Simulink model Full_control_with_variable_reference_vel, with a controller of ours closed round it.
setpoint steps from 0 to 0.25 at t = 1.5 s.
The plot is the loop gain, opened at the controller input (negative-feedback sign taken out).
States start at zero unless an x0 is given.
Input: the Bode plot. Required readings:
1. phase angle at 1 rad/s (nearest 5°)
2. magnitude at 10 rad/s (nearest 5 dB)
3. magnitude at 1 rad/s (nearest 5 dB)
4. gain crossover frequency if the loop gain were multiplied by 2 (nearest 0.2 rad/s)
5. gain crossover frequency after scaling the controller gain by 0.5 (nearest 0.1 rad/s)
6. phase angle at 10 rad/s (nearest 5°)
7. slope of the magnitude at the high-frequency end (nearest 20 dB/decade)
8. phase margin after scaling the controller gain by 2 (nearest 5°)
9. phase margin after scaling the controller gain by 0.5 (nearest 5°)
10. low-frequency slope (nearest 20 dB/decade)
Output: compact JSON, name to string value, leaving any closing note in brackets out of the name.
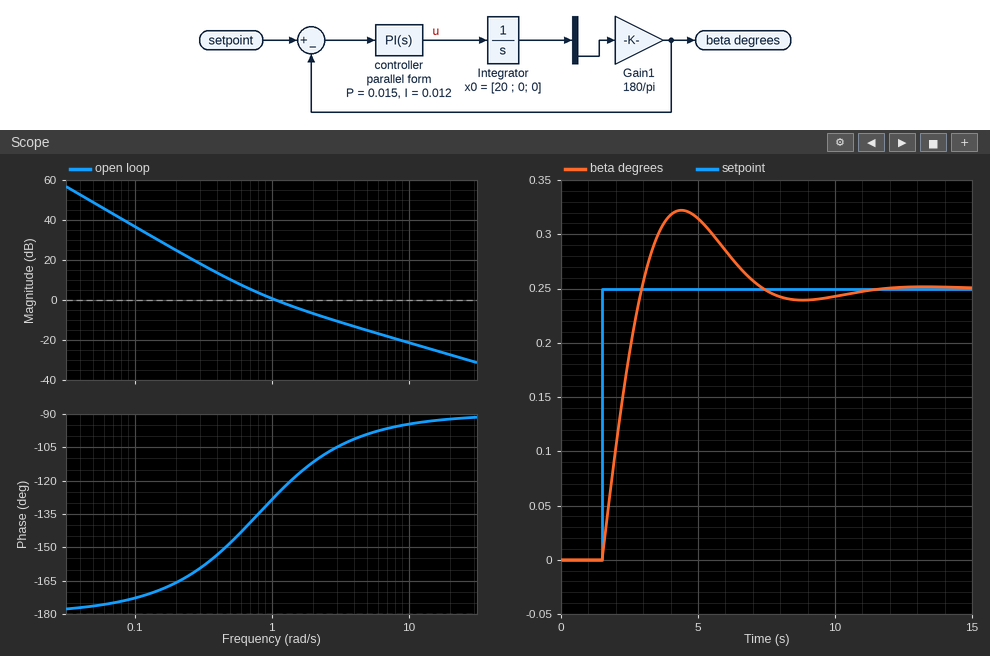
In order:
{"phase angle at 1 rad/s": "-130°", "magnitude at 10 rad/s": "-20 dB", "magnitude at 1 rad/s": "0 dB", "gain crossover frequency if the loop gain were multiplied by 2": "1.8 rad/s", "gain crossover frequency after scaling the controller gain by 0.5": "0.7 rad/s", "phase angle at 10 rad/s": "-95°", "slope of the magnitude at the high-frequency end": "-20 dB/decade", "phase margin after scaling the controller gain by 2": "65°", "phase margin after scaling the controller gain by 0.5": "40°", "low-frequency slope": "-40 dB/decade"}
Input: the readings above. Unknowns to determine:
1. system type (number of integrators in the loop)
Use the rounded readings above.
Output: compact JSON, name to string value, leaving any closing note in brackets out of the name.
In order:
{"system type": "2"}
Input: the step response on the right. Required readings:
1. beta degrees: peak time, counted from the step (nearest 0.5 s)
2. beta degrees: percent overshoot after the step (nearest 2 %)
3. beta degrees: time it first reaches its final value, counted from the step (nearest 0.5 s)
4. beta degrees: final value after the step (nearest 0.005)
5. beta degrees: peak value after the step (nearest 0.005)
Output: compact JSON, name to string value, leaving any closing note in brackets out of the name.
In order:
{"beta degrees: peak time, counted from the step": "3.0 s", "beta degrees: percent overshoot after the step": "28 %", "beta degrees: time it first reaches its final value, counted from the step": "1.5 s", "beta degrees: final value after the step": "0.250", "beta degrees: peak value after the step": "0.320"}
